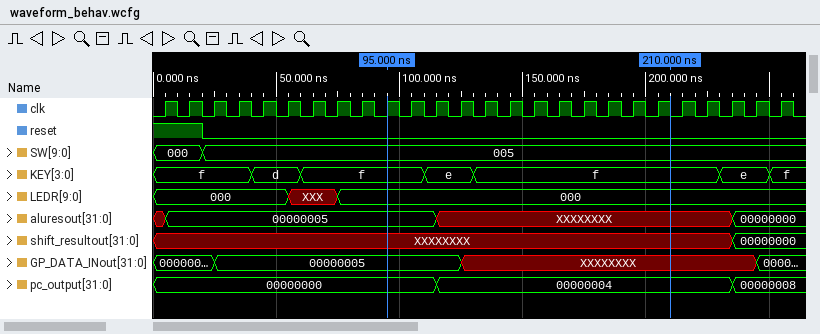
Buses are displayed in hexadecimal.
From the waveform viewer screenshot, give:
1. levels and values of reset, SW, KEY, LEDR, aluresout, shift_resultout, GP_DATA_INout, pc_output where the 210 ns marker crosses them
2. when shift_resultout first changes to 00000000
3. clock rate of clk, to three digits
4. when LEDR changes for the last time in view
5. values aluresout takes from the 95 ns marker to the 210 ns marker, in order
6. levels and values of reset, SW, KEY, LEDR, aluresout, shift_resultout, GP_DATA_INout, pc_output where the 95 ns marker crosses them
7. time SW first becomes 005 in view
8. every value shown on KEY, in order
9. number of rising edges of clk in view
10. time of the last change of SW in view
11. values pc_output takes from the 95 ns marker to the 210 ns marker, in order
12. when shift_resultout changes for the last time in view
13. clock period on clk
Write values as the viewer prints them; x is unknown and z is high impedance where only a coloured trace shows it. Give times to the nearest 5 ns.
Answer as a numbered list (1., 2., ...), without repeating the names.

1. reset=0, SW=005, KEY=f, LEDR=000, aluresout=XXXXXXXX, shift_resultout=XXXXXXXX, GP_DATA_INout=XXXXXXXX, pc_output=00000004
2. 235 ns
3. 100 MHz
4. 75 ns
5. 00000005, XXXXXXXX
6. reset=0, SW=005, KEY=f, LEDR=000, aluresout=00000005, shift_resultout=XXXXXXXX, GP_DATA_INout=00000005, pc_output=00000000
7. 20 ns
8. f, d, f, e, f, e, f
9. 26
10. 20 ns
11. 00000000, 00000004
12. 235 ns
13. 10 ns
